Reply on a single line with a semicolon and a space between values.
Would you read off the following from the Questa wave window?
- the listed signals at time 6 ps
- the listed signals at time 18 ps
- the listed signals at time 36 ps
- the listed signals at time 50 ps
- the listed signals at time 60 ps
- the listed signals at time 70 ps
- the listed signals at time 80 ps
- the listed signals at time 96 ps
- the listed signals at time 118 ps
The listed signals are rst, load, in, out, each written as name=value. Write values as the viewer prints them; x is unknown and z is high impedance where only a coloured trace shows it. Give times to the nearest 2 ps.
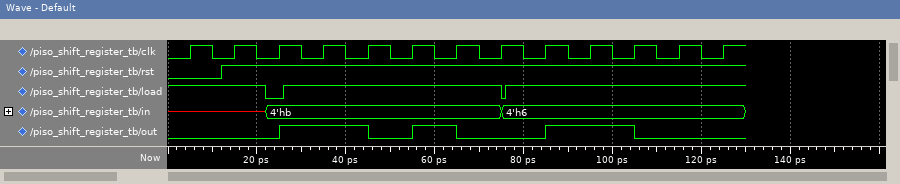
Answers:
rst=0, load=1, in=x, out=0; rst=1, load=1, in=x, out=0; rst=1, load=1, in=4'hb, out=1; rst=1, load=1, in=4'hb, out=0; rst=1, load=1, in=4'hb, out=1; rst=1, load=1, in=4'hb, out=0; rst=1, load=1, in=4'h6, out=0; rst=1, load=1, in=4'h6, out=1; rst=1, load=1, in=4'h6, out=0
